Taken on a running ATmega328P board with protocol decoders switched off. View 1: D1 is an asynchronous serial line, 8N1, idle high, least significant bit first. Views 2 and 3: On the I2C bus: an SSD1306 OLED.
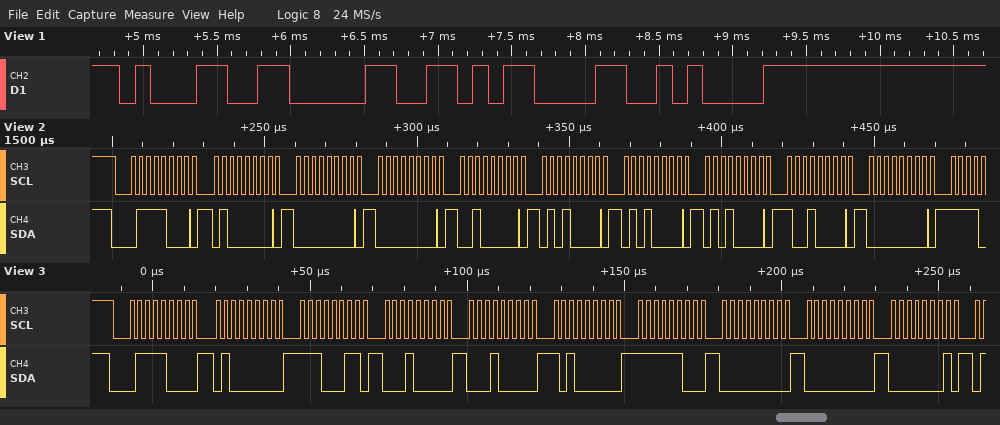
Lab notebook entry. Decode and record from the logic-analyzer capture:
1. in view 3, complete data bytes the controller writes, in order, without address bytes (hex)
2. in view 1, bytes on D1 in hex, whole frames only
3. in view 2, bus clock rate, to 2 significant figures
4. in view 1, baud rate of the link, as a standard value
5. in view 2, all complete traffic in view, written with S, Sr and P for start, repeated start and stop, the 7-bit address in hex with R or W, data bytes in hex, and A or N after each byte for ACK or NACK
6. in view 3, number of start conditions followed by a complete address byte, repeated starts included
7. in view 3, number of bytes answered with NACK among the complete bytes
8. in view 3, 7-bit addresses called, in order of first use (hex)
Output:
40 E3 10 10 A0 FC 00 00 01
31 30 0D 0A
400 kHz
9600 baud
S 3CW A 40 A 00 A 00 A 20 A 50 A 50 A 50 A 90 A 00 A
1
0
0x3C
